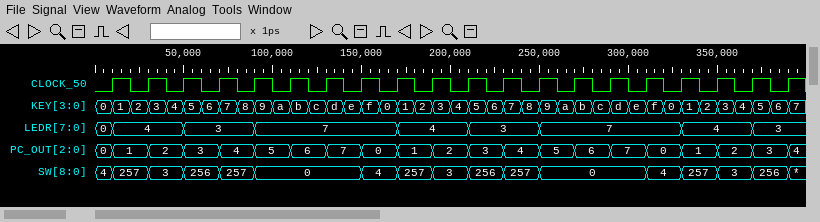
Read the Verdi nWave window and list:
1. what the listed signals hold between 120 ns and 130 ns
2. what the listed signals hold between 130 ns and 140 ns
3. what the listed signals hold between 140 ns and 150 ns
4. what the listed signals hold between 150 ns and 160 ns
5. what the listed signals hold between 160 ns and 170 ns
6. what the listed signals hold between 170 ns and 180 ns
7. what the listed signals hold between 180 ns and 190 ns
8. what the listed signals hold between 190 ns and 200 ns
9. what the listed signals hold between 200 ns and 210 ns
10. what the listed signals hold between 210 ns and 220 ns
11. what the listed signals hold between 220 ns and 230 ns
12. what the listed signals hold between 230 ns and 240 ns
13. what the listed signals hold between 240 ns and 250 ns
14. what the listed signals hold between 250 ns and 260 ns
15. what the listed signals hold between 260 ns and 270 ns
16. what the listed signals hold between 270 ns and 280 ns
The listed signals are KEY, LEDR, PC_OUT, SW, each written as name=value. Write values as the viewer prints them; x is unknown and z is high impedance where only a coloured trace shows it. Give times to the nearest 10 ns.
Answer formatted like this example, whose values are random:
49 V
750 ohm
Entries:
KEY=c, LEDR=7, PC_OUT=6, SW=0
KEY=d, LEDR=7, PC_OUT=7, SW=0
KEY=e, LEDR=7, PC_OUT=7, SW=0
KEY=f, LEDR=7, PC_OUT=0, SW=4
KEY=0, LEDR=7, PC_OUT=0, SW=4
KEY=1, LEDR=4, PC_OUT=1, SW=257
KEY=2, LEDR=4, PC_OUT=1, SW=257
KEY=3, LEDR=4, PC_OUT=2, SW=3
KEY=4, LEDR=4, PC_OUT=2, SW=3
KEY=5, LEDR=3, PC_OUT=3, SW=256
KEY=6, LEDR=3, PC_OUT=3, SW=256
KEY=7, LEDR=3, PC_OUT=4, SW=257
KEY=8, LEDR=3, PC_OUT=4, SW=257
KEY=9, LEDR=7, PC_OUT=5, SW=0
KEY=a, LEDR=7, PC_OUT=5, SW=0
KEY=b, LEDR=7, PC_OUT=6, SW=0
